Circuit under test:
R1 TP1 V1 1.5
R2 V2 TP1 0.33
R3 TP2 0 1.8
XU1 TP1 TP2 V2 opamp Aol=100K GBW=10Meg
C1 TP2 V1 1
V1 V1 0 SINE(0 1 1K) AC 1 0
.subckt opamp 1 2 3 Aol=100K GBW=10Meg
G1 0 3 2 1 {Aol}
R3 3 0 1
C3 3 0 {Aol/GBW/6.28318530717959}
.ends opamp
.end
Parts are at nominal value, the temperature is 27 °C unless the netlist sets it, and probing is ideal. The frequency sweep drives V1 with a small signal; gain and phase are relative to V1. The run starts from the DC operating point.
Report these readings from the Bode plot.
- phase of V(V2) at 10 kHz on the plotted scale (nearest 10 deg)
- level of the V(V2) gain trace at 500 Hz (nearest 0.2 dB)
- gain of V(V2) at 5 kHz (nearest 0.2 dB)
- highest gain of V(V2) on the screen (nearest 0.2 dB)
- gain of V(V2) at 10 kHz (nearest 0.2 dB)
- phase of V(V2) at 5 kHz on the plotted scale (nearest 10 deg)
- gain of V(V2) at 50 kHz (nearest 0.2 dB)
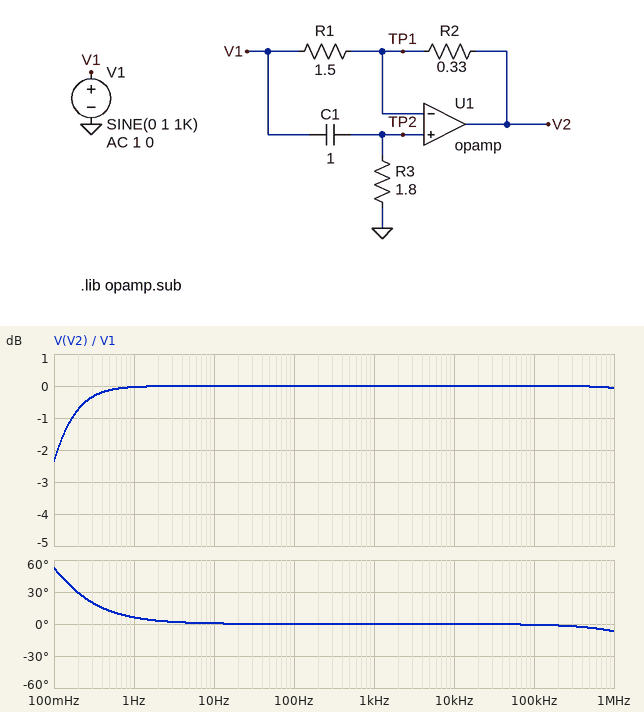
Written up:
0 deg
0 dB
0 dB
0 dB
0 dB
0 deg
0 dB
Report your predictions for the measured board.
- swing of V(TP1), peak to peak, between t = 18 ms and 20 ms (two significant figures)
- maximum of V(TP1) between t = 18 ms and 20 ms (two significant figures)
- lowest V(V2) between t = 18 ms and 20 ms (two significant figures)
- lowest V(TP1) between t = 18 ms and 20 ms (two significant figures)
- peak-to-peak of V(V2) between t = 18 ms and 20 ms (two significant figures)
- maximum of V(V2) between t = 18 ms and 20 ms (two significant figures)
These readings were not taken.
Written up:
2.0 V
1.0 V
-1.0 V
-1.0 V
2.0 V
1.0 V
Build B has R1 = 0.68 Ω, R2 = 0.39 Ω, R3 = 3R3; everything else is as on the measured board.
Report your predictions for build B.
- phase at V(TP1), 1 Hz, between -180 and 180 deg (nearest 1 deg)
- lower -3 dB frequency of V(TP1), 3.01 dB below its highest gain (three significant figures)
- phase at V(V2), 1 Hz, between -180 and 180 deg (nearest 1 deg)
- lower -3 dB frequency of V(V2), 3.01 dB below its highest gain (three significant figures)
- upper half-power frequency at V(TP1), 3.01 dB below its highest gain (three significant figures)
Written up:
3 deg
48.2 mHz
4 deg
28.2 mHz
7.42 MHz
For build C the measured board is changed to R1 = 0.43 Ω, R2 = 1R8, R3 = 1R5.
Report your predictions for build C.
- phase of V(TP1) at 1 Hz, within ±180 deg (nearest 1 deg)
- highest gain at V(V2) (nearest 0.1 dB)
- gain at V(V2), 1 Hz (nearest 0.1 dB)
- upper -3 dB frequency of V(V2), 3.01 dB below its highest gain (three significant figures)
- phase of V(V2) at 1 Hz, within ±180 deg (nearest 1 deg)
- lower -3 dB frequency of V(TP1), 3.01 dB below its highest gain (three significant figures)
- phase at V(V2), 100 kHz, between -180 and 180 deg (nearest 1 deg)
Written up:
6 deg
12.4 dB
0.7 dB
113 mHz
30 deg
106 mHz
-3 deg
